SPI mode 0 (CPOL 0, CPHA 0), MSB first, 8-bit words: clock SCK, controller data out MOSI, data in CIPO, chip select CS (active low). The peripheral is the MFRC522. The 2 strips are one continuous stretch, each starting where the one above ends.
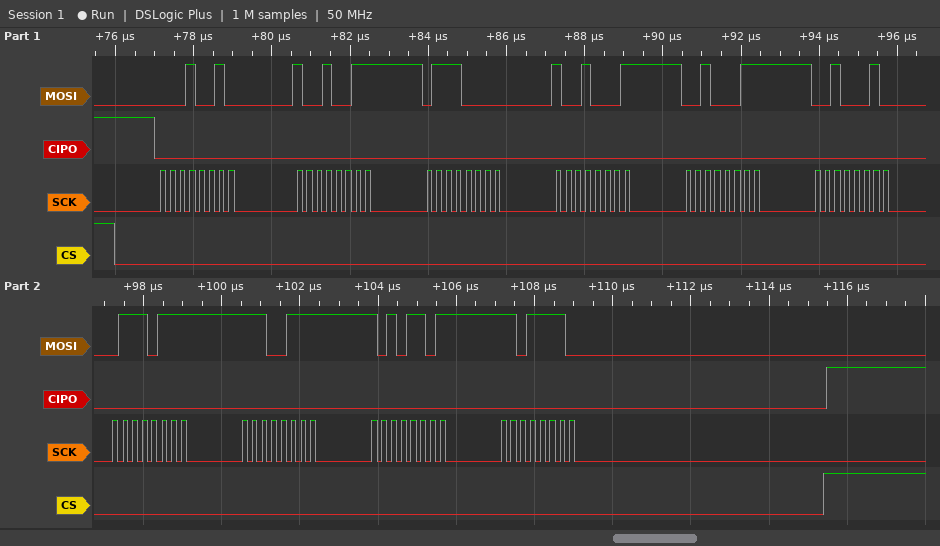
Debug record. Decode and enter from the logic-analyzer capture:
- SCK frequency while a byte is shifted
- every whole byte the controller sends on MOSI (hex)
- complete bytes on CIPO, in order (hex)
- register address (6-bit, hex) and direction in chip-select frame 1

4 MHz
0x12 0x93 0x70 0x91 0x23 0x22 0x77 0xE7 0xAD 0xDE
0x00 0x00 0x00 0x00 0x00 0x00 0x00 0x00 0x00 0x00
0x09 write
